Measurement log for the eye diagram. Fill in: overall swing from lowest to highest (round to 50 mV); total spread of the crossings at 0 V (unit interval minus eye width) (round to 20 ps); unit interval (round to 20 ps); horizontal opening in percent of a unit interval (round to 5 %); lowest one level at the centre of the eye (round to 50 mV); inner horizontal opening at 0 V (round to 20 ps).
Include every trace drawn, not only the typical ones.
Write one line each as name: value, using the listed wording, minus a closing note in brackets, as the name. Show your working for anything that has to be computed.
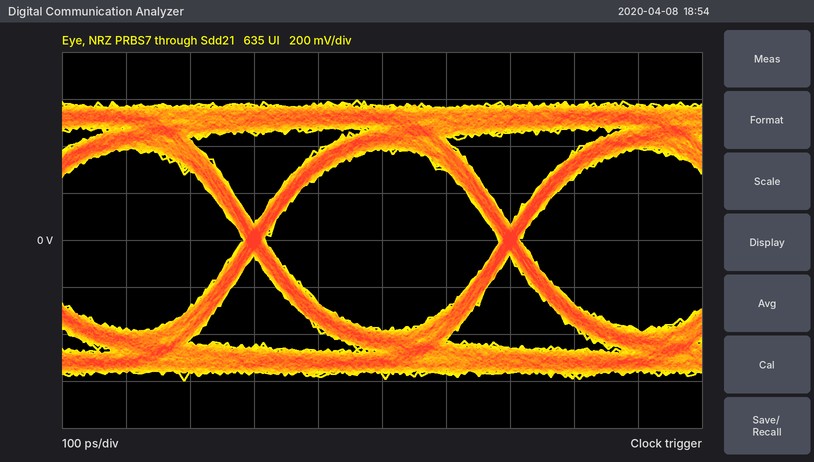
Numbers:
overall swing from lowest to highest: 1.20 V
total spread of the crossings at 0 V (unit interval minus eye width): 40 ps
unit interval: 400 ps
horizontal opening in percent of a unit interval: 360 ps / 400 ps ≈ 90 %
lowest one level at the centre of the eye: 400 mV
inner horizontal opening at 0 V: 360 ps
